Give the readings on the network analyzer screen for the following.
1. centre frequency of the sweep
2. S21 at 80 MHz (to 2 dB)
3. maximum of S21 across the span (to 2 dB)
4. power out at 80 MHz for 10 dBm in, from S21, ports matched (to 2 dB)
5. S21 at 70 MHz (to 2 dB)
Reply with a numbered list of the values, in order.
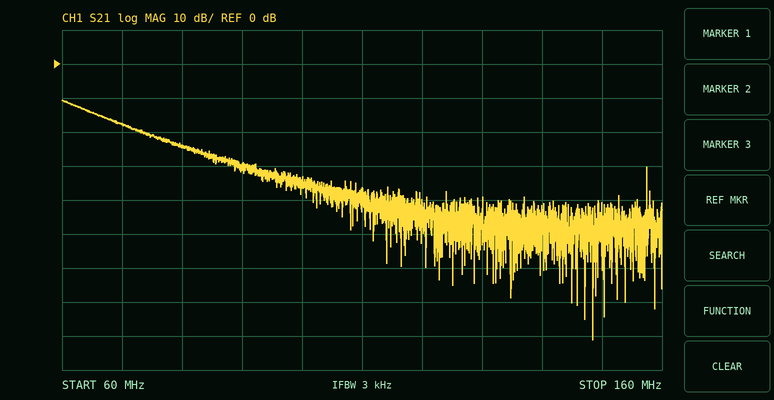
1. 110 MHz
2. -24 dB
3. -10 dB
4. -14 dBm
5. -18 dB
